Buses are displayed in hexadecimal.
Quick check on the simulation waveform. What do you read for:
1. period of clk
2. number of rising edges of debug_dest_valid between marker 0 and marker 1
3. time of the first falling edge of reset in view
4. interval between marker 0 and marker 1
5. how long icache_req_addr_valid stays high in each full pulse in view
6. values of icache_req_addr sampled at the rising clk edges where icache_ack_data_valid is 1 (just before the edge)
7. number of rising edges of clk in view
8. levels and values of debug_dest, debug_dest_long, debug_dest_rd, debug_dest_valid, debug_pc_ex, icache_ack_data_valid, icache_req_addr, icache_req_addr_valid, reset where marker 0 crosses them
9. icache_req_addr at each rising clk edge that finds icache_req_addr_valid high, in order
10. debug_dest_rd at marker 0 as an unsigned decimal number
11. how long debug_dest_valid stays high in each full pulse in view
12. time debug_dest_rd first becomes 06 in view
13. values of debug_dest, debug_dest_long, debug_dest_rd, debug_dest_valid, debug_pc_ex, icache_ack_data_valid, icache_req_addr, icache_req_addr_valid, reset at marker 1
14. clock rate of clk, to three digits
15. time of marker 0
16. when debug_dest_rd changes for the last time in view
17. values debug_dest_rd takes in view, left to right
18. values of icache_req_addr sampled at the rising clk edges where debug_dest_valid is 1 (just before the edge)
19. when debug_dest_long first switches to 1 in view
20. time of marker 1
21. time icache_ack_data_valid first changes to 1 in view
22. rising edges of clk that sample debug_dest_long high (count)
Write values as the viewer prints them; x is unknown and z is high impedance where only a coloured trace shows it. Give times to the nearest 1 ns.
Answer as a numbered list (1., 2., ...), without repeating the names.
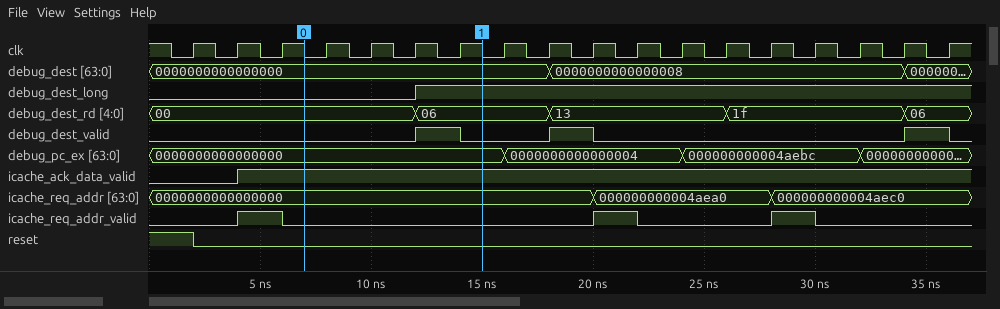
1. 2 ns
2. 1
3. 2 ns
4. 8 ns
5. 2 ns, 2 ns, 2 ns
6. 0000000000000000, 0000000000000000, 0000000000000000, 0000000000000000, 0000000000000000, 0000000000000000, 0000000000000000, 0000000000000000, 000000000004aea0, 000000000004aea0, 000000000004aea0, 000000000004aea0, 000000000004aec0, 000000000004aec0, 000000000004aec0, 000000000004aec0
7. 18
8. debug_dest=0000000000000000, debug_dest_long=0, debug_dest_rd=00, debug_dest_valid=0, debug_pc_ex=0000000000000000, icache_ack_data_valid=1, icache_req_addr=0000000000000000, icache_req_addr_valid=0, reset=0
9. 0000000000000000, 000000000004aea0, 000000000004aec0
10. 0
11. 2 ns, 2 ns, 2 ns
12. 12 ns
13. debug_dest=0000000000000000, debug_dest_long=1, debug_dest_rd=06, debug_dest_valid=0, debug_pc_ex=0000000000000000, icache_ack_data_valid=1, icache_req_addr=0000000000000000, icache_req_addr_valid=0, reset=0
14. 500 MHz
15. 7 ns
16. 34 ns
17. 00, 06, 13, 1f, 06
18. 0000000000000000, 0000000000000000, 000000000004aec0
19. 12 ns
20. 15 ns
21. 4 ns
22. 12
